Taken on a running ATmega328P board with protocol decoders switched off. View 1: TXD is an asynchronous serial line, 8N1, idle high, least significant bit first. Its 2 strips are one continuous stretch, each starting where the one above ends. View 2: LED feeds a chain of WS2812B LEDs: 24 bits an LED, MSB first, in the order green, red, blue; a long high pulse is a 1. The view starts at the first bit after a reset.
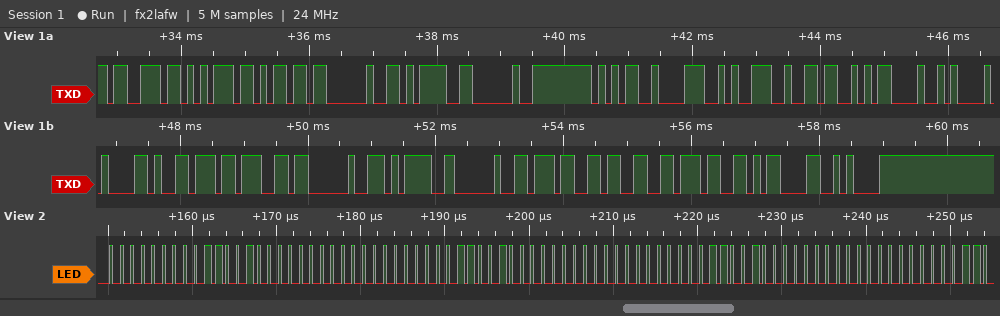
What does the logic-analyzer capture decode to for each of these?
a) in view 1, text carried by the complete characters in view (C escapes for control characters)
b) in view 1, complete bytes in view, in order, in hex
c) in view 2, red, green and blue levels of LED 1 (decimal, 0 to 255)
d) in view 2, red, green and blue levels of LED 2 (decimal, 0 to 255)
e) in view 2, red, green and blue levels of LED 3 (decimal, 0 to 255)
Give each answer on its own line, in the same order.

"sum = 5896\r\navg = 737\r\n"
73 75 6D 20 3D 20 35 38 39 36 0D 0A 61 76 67 20 3D 20 37 33 37 0D 0A
100, 0, 0
100, 0, 0
100, 0, 0
